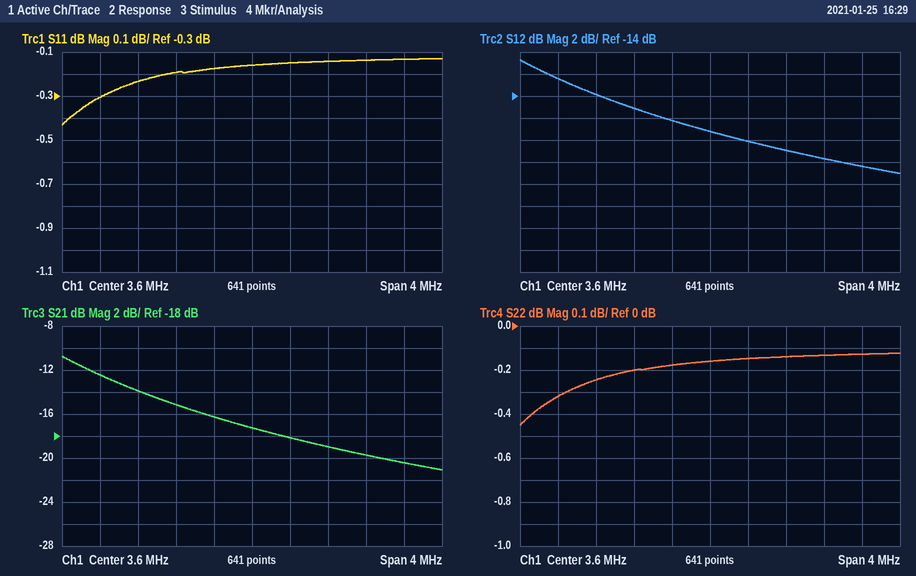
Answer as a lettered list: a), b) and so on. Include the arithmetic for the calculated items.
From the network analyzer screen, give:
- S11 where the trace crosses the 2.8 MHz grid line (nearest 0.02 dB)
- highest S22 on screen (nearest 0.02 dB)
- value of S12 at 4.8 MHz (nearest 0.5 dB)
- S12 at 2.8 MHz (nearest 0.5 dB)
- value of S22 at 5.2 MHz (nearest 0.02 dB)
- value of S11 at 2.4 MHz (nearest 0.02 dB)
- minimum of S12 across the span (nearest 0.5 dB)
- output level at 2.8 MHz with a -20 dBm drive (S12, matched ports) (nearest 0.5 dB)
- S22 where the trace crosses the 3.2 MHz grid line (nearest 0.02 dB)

a) -0.20 dB
b) -0.12 dB
c) -19.5 dB
d) -15.0 dB
e) -0.12 dB
f) -0.24 dB
g) -21.0 dB
h) -20 dBm + (-15.0 dB) = -35.0 dBm
i) -0.18 dB
